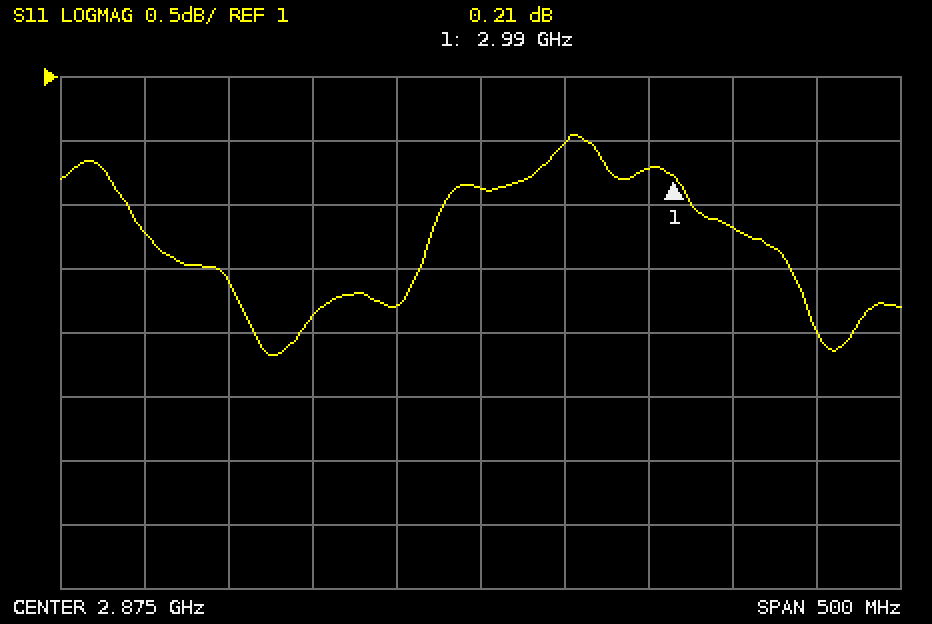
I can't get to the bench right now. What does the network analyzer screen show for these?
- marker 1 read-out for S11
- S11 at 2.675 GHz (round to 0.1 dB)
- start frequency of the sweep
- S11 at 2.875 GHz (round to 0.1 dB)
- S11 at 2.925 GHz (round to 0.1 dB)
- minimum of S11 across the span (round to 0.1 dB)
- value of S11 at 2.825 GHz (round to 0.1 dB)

0.21 dB
-0.2 dB
2.625 GHz
0.1 dB
0.5 dB
-1.2 dB
-0.8 dB
